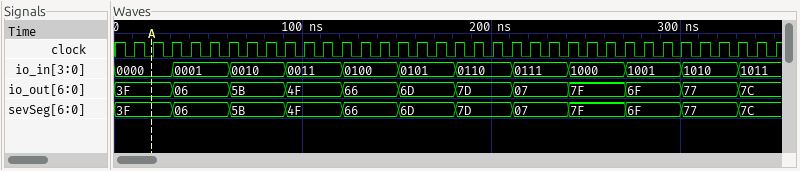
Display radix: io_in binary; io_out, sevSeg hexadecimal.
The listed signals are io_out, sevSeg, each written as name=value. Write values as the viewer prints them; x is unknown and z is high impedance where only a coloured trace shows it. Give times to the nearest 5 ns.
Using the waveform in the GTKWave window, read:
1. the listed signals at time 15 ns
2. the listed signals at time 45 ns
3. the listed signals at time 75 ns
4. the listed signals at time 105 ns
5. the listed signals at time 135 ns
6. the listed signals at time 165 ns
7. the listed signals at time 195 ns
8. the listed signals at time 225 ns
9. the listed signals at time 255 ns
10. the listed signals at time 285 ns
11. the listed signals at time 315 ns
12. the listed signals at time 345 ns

io_out=3F, sevSeg=3F
io_out=06, sevSeg=06
io_out=5B, sevSeg=5B
io_out=4F, sevSeg=4F
io_out=66, sevSeg=66
io_out=6D, sevSeg=6D
io_out=7D, sevSeg=7D
io_out=07, sevSeg=07
io_out=7F, sevSeg=7F
io_out=6F, sevSeg=6F
io_out=77, sevSeg=77
io_out=7C, sevSeg=7C
